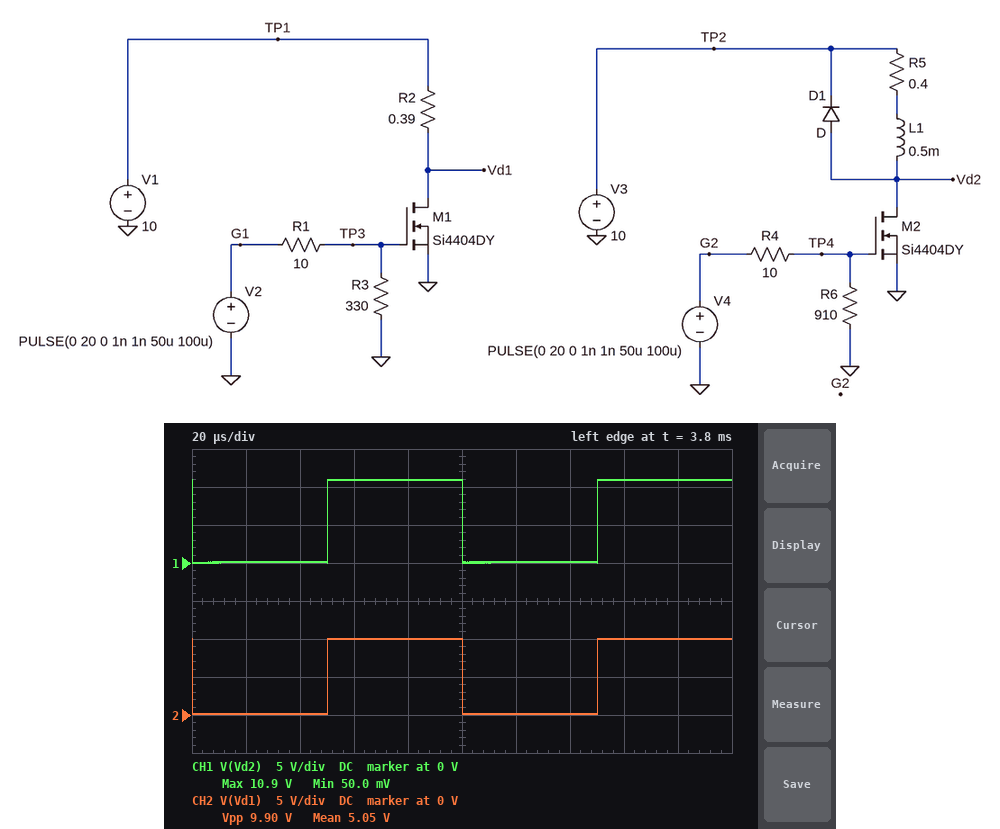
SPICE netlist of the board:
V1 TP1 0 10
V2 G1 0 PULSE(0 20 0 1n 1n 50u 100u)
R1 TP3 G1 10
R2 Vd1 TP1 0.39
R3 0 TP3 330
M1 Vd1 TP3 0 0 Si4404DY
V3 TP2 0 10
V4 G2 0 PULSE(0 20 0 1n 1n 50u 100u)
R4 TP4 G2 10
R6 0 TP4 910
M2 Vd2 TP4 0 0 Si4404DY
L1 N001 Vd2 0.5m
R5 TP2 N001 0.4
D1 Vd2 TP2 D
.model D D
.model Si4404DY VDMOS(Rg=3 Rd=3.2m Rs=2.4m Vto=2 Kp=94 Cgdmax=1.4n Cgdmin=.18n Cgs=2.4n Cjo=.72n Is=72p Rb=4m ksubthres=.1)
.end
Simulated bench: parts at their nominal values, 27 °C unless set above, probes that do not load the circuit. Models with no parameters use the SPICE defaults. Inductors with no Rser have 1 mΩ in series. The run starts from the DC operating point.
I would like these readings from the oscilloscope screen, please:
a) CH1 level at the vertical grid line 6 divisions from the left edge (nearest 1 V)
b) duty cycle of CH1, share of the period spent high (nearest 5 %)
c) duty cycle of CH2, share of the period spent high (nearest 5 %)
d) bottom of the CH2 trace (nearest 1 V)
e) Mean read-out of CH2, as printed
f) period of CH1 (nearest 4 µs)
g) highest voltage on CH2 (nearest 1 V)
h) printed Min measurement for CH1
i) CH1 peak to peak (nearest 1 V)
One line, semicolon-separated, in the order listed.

0 V; 50 %; 50 %; 0 V; 5.05 V; 100 µs; 10 V; 50.0 mV; 11 V
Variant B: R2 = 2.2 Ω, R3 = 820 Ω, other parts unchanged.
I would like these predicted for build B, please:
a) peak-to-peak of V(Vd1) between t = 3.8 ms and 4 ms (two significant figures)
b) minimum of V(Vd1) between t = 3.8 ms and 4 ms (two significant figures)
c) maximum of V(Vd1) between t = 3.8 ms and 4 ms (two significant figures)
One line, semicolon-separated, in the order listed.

10 V; 24 mV; 10 V
